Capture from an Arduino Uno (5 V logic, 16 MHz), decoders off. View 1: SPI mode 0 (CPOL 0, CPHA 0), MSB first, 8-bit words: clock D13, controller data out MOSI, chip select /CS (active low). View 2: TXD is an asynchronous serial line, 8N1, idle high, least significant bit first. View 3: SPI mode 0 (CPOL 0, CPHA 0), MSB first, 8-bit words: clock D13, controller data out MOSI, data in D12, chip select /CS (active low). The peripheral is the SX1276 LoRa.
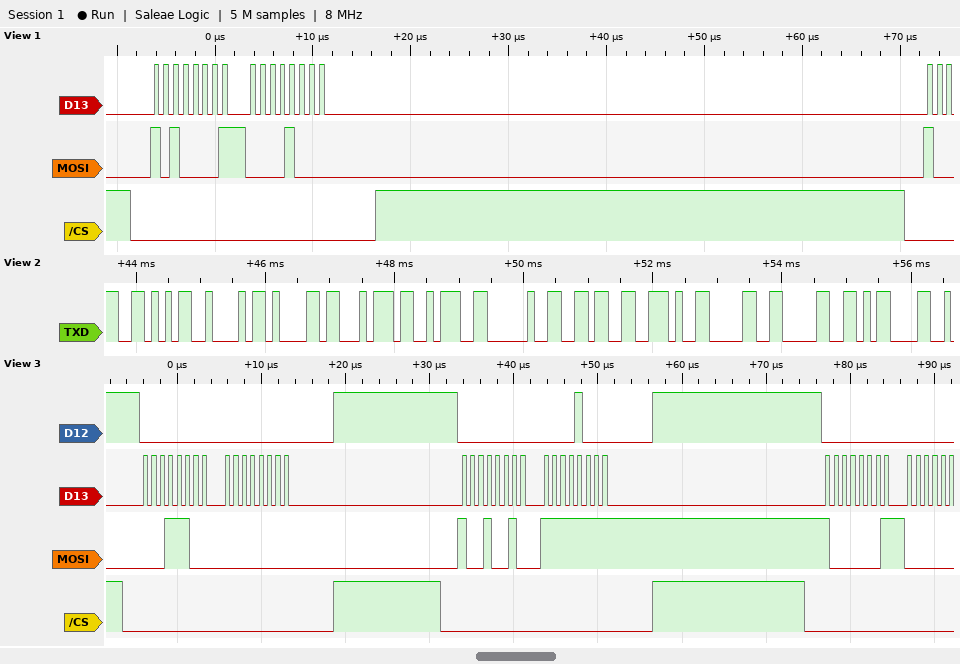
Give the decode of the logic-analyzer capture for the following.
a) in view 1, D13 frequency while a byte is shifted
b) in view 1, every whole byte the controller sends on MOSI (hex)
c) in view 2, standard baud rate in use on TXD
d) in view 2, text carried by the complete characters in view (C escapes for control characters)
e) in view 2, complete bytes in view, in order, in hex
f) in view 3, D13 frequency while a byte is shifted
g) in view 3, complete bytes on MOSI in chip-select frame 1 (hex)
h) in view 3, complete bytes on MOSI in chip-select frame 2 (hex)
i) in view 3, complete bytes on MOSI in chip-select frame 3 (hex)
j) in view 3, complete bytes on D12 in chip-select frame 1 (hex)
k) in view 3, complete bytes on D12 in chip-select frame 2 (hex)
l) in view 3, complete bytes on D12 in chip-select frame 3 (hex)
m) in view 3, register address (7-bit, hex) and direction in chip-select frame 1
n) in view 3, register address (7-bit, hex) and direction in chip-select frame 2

1 MHz
0xA1 0x08
9600 baud
"VBat: 6.00\r"
56 42 61 74 3A 20 36 2E 30 30 0D
1 MHz
1C 00
92 FF
81
00 00
00 08
00
0x1C read
0x12 write
